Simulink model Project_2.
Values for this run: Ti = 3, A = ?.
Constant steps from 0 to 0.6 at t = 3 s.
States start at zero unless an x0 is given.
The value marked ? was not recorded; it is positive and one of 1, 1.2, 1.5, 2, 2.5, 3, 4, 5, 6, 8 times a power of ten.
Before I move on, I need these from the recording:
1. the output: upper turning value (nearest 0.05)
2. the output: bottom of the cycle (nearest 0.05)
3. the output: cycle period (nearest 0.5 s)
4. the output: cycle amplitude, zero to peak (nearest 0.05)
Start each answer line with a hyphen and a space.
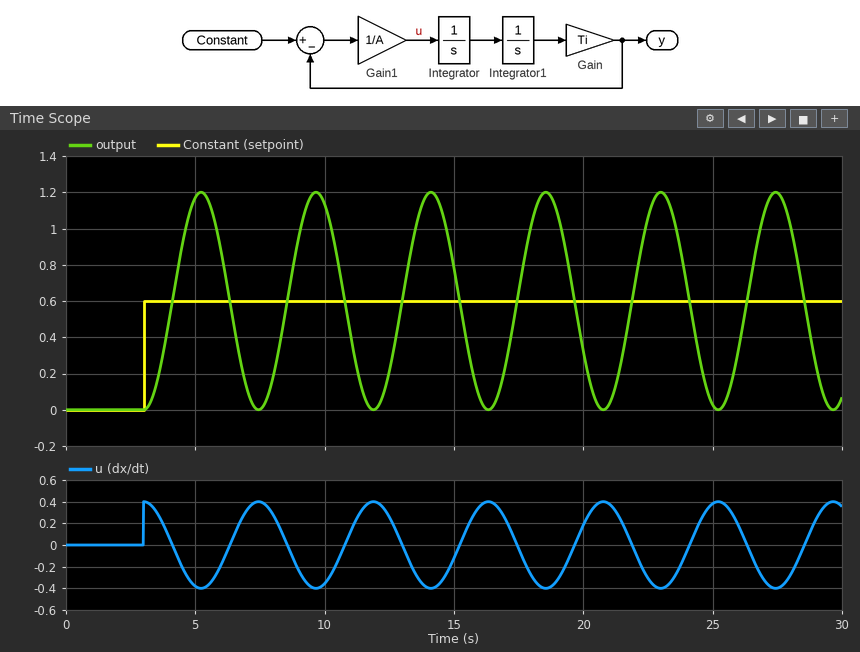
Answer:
- 1.20
- 0.00
- 4.5 s
- 0.60
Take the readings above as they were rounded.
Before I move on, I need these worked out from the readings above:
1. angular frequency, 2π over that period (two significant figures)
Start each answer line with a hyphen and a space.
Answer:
- 1.4 rad/s
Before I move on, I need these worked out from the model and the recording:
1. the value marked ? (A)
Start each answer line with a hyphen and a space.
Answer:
- 1.5
